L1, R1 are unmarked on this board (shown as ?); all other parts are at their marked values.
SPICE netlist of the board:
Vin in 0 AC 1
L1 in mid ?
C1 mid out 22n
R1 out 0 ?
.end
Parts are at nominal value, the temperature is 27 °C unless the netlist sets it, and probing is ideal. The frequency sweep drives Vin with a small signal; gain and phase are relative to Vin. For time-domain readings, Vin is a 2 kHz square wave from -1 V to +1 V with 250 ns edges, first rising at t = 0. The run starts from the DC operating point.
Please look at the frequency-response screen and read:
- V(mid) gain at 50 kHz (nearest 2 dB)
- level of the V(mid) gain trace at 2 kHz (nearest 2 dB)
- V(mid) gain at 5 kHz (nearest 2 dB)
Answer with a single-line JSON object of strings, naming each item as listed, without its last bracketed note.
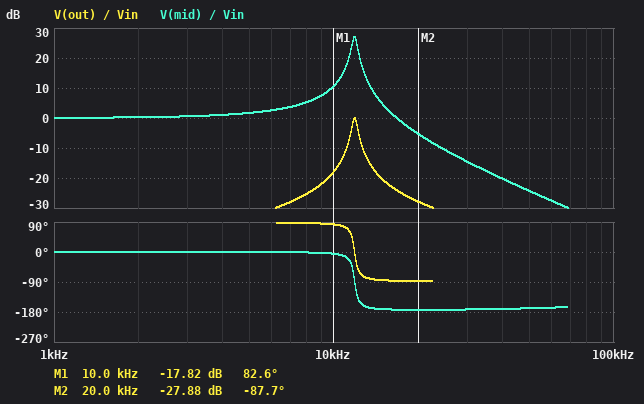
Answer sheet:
{"V(mid) gain at 50 kHz": "-24 dB", "level of the V(mid) gain trace at 2 kHz": "0 dB", "V(mid) gain at 5 kHz": "2 dB"}
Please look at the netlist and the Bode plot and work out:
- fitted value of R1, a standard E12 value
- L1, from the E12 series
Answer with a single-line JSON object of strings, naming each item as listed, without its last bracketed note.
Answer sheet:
{"fitted value of R1, a standard E12 value": "27 Ω", "L1, from the E12 series": "8.2 mH"}
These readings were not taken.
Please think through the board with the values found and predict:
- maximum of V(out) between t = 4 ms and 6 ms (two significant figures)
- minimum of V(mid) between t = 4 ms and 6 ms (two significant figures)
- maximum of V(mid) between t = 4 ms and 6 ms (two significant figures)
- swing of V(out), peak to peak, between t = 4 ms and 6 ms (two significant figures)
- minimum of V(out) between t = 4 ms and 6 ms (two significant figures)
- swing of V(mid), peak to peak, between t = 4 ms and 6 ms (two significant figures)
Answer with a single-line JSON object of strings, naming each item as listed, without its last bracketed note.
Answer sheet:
{"maximum of V(out) between t = 4 ms and 6 ms": "52 mV", "minimum of V(mid) between t = 4 ms and 6 ms": "-2.1 V", "maximum of V(mid) between t = 4 ms and 6 ms": "2.1 V", "swing of V(out), peak to peak, between t = 4 ms and 6 ms": "100 mV", "minimum of V(out) between t = 4 ms and 6 ms": "-52 mV", "swing of V(mid), peak to peak, between t = 4 ms and 6 ms": "4.3 V"}
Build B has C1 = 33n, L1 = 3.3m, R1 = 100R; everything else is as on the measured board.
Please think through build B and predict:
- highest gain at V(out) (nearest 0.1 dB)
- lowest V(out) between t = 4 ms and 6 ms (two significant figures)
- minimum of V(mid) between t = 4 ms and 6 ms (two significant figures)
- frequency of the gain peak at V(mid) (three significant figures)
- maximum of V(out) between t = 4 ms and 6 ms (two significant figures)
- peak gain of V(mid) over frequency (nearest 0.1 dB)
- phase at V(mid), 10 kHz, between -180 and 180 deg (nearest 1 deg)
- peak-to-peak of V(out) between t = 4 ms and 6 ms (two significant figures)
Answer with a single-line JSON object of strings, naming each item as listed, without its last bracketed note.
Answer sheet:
{"highest gain at V(out)": "0 dB", "lowest V(out) between t = 4 ms and 6 ms": "-510 mV", "minimum of V(mid) between t = 4 ms and 6 ms": "-2.3 V", "frequency of the gain peak at V(mid)": "14.9 kHz", "maximum of V(out) between t = 4 ms and 6 ms": "510 mV", "peak gain of V(mid) over frequency": "10.5 dB", "phase at V(mid), 10 kHz, between -180 and 180 deg": "-8 deg", "peak-to-peak of V(out) between t = 4 ms and 6 ms": "1.0 V"}
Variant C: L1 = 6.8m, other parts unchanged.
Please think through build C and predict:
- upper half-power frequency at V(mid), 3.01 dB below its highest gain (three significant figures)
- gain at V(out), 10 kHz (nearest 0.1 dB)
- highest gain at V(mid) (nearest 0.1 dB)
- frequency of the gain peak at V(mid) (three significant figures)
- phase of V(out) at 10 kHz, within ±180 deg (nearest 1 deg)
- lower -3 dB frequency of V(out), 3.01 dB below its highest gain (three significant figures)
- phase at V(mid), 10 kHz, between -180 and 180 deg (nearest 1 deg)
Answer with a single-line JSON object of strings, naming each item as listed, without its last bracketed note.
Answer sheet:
{"upper half-power frequency at V(mid), 3.01 dB below its highest gain": "13.3 kHz", "gain at V(out), 10 kHz": "-20.8 dB", "highest gain at V(mid)": "26.3 dB", "frequency of the gain peak at V(mid)": "13.0 kHz", "phase of V(out) at 10 kHz, within ±180 deg": "85 deg", "lower -3 dB frequency of V(out), 3.01 dB below its highest gain": "12.7 kHz", "phase at V(mid), 10 kHz, between -180 and 180 deg": "-3 deg"}
